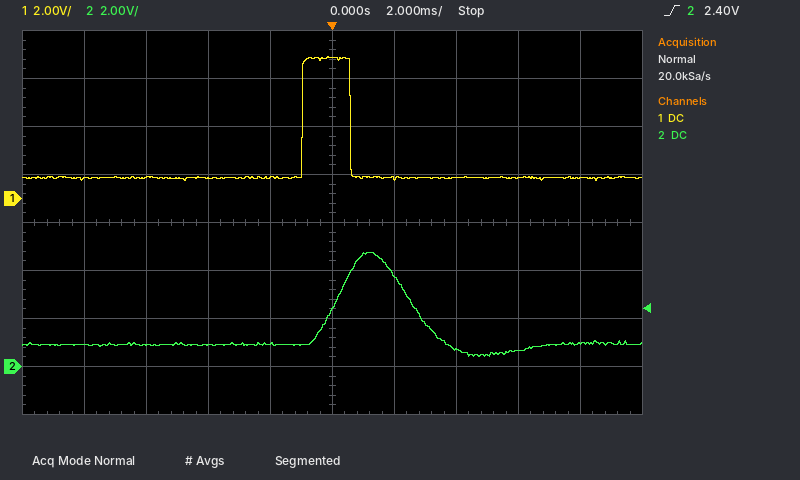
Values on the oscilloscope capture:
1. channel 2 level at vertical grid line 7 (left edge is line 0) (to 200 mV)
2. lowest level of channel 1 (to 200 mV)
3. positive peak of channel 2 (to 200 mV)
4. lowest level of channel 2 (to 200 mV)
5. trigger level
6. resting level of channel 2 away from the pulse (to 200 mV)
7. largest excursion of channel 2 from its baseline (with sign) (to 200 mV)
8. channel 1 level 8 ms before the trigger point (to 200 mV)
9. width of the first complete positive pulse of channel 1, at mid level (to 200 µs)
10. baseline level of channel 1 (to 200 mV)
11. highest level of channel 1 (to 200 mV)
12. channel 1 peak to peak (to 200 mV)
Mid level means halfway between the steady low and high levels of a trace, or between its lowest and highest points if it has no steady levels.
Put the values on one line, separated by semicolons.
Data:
800 mV; 800 mV; 4.8 V; 400 mV; 2.40 V; 1.0 V; +3.8 V; 800 mV; 1.6 ms; 800 mV; 6.0 V; 5.2 V
